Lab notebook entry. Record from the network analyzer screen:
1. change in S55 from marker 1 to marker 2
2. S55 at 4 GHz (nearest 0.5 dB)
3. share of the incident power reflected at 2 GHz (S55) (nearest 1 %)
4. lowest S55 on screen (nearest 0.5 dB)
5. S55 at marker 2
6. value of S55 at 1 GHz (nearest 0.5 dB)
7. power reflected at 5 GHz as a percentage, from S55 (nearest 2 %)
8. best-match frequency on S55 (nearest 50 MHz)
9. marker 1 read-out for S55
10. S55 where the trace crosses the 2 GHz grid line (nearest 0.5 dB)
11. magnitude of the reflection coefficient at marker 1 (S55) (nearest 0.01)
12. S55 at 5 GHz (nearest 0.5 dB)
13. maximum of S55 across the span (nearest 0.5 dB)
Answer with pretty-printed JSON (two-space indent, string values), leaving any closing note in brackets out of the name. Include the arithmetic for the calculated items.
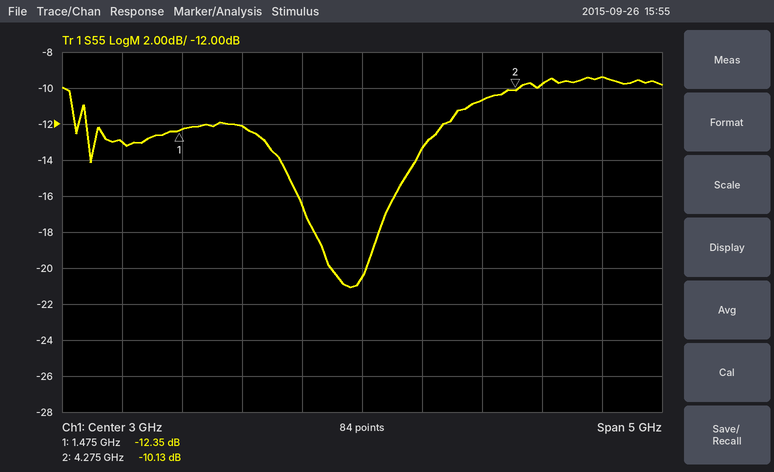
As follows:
{
  "change in S55 from marker 1 to marker 2": "-10.13 − (-12.35) = 2.22 dB",
  "S55 at 4 GHz": "-10.5 dB",
  "share of the incident power reflected at 2 GHz (S55)": "10^(-12/10) ≈ 6 %",
  "lowest S55 on screen": "-21.0 dB",
  "S55 at marker 2": "-10.13 dB",
  "value of S55 at 1 GHz": "-13.0 dB",
  "power reflected at 5 GHz as a percentage, from S55": "10^(-9.5/10) ≈ 11.2 %, so 12 % to the nearest 2 %",
  "best-match frequency on S55": "2.90 GHz",
  "marker 1 read-out for S55": "-12.35 dB",
  "S55 where the trace crosses the 2 GHz grid line": "-12.0 dB",
  "magnitude of the reflection coefficient at marker 1 (S55)": "10^(-12.35/20) ≈ 0.24",
  "S55 at 5 GHz": "-9.5 dB",
  "maximum of S55 across the span": "-9.5 dB"
}
